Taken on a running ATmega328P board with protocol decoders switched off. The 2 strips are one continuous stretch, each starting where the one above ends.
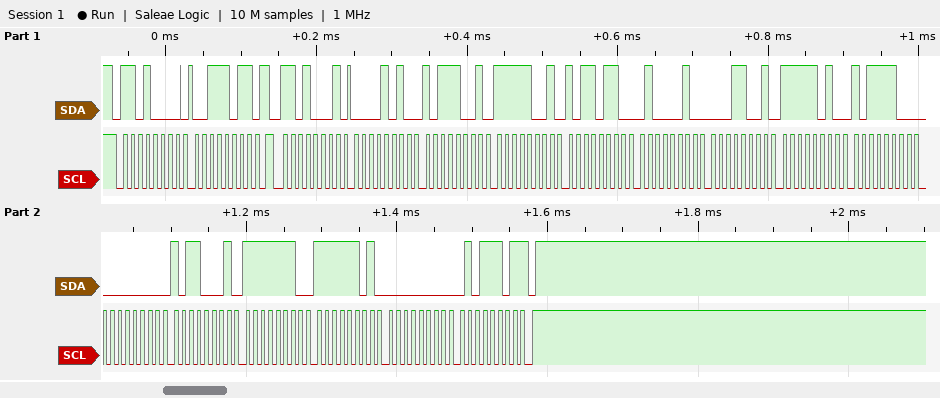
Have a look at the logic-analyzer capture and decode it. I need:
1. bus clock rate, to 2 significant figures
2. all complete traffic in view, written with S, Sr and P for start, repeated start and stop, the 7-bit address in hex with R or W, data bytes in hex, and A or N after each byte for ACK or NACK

100 kHz
S 68W A 3B A Sr 68R A 0A A B9 A F9 A B6 A 42 A 19 A FA A BC A 00 A B1 A FE A FD A 00 A 5D N P
